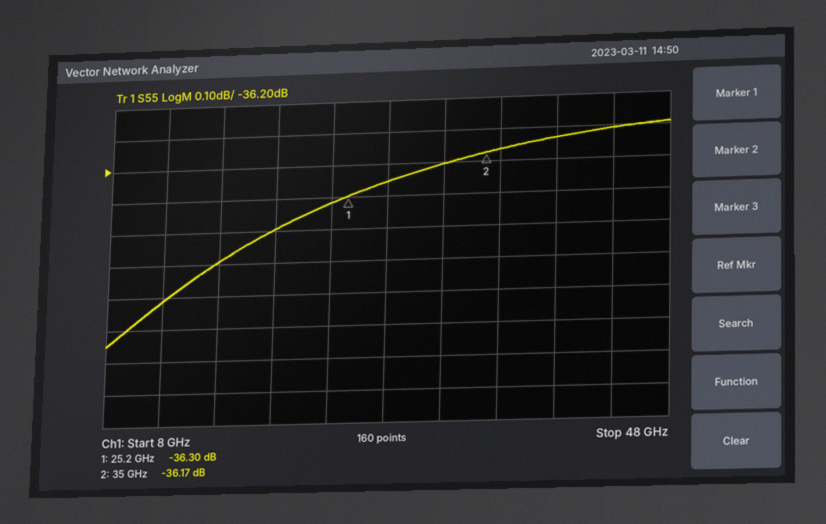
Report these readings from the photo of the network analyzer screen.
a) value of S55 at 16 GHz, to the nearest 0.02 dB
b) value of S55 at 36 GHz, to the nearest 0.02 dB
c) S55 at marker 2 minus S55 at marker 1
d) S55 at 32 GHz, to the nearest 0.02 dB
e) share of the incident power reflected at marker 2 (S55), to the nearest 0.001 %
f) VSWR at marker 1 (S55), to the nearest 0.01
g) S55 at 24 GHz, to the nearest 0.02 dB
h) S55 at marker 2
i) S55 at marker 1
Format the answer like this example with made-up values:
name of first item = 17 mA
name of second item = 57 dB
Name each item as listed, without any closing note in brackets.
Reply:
value of S55 at 16 GHz, to the nearest 0.02 dB = -36.50 dB
value of S55 at 36 GHz, to the nearest 0.02 dB = -36.16 dB
S55 at marker 2 minus S55 at marker 1 = 0.13 dB
S55 at 32 GHz, to the nearest 0.02 dB = -36.20 dB
share of the incident power reflected at marker 2 (S55), to the nearest 0.001 % = 0.024 %
VSWR at marker 1 (S55), to the nearest 0.01 = 1.03
S55 at 24 GHz, to the nearest 0.02 dB = -36.32 dB
S55 at marker 2 = -36.17 dB
S55 at marker 1 = -36.30 dB
